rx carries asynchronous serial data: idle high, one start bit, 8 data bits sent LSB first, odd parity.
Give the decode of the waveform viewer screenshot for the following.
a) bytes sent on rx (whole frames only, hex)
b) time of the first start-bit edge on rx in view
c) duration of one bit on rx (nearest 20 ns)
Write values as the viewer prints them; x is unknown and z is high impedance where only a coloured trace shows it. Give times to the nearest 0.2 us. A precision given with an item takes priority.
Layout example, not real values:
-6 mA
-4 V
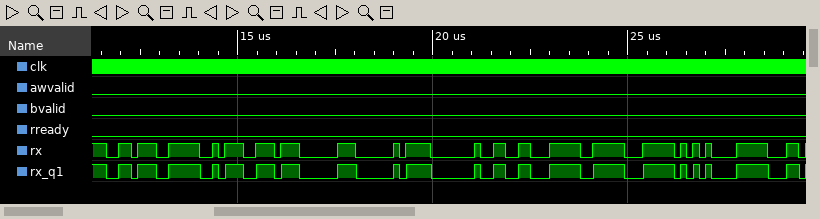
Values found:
76, 3A, 07, A0, 40, C6, 3E, 15
11.6 us
160 ns
